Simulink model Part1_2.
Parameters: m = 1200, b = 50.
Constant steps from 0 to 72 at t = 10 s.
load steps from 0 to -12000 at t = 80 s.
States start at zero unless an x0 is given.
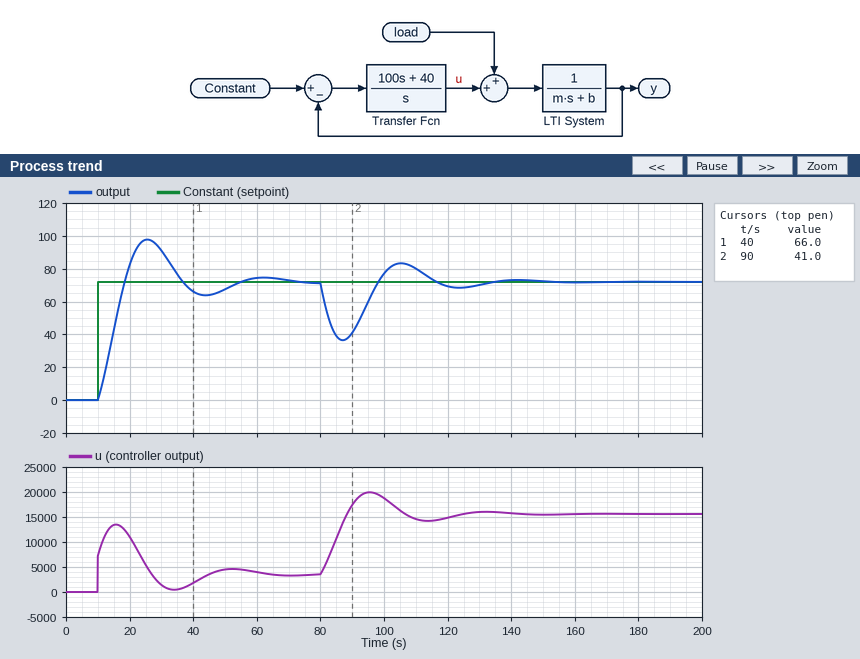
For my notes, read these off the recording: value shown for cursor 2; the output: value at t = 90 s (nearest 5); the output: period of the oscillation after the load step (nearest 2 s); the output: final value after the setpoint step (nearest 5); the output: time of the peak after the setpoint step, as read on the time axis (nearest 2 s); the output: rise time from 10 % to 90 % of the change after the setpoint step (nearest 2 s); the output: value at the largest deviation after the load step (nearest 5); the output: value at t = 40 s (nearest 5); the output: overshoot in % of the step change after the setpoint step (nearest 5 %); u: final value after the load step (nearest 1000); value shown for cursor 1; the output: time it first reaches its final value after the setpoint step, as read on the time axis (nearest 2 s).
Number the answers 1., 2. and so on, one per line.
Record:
1. 41.0
2. 40
3. 36 s
4. 70
5. 26 s
6. 6 s
7. 35
8. 65
9. 35 %
10. 16000
11. 66.0
12. 18 s
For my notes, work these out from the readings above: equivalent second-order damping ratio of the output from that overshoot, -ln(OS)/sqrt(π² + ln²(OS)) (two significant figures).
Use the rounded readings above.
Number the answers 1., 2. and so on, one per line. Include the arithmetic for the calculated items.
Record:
1. ln(0.35) = -1.050; 1.050 / sqrt(9.870 + 1.102) = 0.32
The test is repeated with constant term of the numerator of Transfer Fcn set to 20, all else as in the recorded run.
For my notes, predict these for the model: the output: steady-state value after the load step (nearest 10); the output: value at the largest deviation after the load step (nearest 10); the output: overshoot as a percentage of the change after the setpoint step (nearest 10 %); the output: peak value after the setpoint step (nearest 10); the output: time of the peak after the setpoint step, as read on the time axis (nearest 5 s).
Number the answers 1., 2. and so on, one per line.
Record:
1. 70
2. 30
3. 20 %
4. 90
5. 30 s
